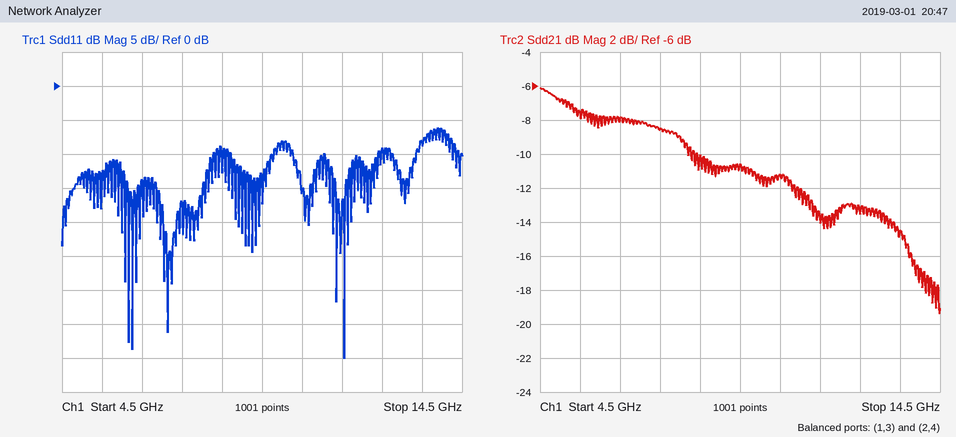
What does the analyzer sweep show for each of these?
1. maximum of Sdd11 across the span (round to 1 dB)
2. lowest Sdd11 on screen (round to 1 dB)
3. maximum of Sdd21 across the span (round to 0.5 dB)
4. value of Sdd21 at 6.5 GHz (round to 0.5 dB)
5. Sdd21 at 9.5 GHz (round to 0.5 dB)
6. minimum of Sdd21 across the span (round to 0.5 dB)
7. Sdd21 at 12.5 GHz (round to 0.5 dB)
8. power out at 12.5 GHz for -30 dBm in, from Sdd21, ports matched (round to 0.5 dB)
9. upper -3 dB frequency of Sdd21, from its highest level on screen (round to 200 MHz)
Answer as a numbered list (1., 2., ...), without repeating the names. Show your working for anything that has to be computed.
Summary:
1. -6 dB
2. -40 dB
3. -6.0 dB
4. -8.0 dB
5. -10.5 dB
6. -19.5 dB
7. -13.5 dB
8. -30 dBm + (-13.5 dB) = -43.5 dBm
9. 8.0 GHz
